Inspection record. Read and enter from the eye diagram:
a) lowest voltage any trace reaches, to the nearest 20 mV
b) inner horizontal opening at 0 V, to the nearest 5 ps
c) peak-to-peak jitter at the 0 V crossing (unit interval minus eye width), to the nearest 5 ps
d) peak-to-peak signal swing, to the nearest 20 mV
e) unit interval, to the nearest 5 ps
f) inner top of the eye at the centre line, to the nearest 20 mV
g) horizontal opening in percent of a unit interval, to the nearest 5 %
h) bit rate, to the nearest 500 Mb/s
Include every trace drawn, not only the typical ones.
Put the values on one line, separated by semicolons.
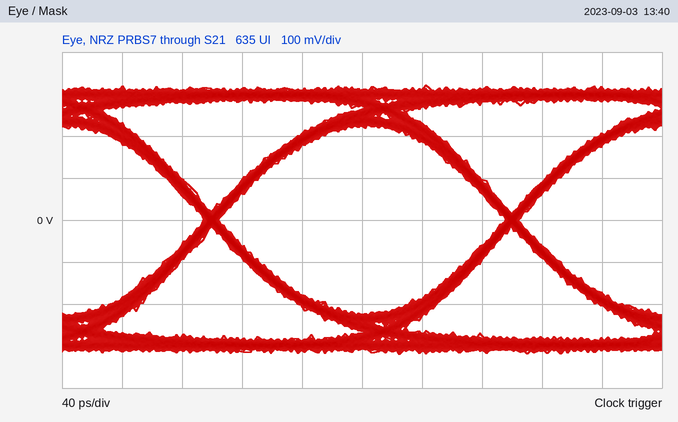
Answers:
-320 mV; 190 ps; 10 ps; 640 mV; 200 ps; 220 mV; 95 %; 5.0 Gb/s
